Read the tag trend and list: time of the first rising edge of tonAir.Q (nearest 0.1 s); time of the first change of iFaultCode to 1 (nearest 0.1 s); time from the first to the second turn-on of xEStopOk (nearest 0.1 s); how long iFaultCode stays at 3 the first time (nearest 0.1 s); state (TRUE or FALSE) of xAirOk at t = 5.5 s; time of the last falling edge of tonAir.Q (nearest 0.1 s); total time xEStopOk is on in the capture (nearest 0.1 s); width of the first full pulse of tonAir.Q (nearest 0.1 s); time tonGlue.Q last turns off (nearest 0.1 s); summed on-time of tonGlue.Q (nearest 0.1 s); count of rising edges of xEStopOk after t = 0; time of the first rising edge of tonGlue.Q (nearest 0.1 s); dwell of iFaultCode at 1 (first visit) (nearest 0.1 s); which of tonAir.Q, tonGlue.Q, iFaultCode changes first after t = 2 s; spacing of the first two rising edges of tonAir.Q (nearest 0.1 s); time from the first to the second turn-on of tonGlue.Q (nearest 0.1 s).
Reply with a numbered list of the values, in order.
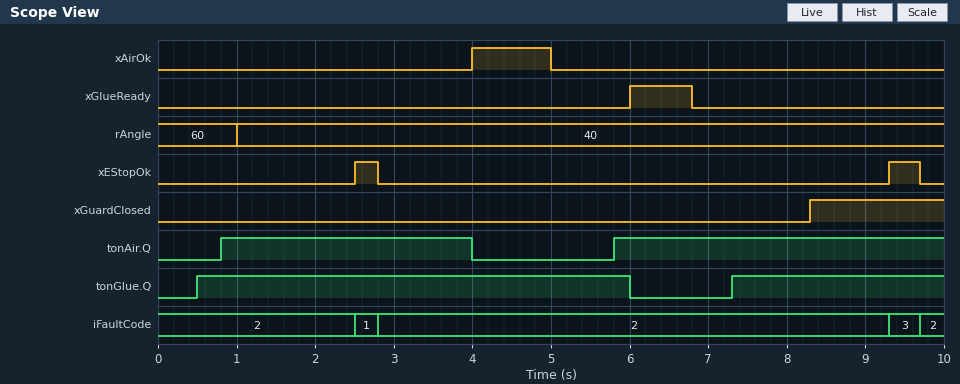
1. 0.8 s
2. 2.5 s
3. 6.8 s
4. 0.4 s
5. FALSE
6. 4.0 s
7. 0.7 s
8. 3.2 s
9. 6.0 s
10. 8.2 s
11. 2
12. 0.5 s
13. 0.3 s
14. iFaultCode
15. 5.0 s
16. 6.8 s
